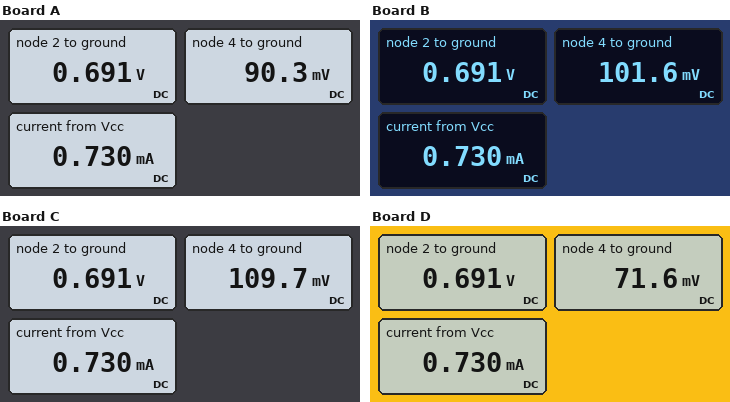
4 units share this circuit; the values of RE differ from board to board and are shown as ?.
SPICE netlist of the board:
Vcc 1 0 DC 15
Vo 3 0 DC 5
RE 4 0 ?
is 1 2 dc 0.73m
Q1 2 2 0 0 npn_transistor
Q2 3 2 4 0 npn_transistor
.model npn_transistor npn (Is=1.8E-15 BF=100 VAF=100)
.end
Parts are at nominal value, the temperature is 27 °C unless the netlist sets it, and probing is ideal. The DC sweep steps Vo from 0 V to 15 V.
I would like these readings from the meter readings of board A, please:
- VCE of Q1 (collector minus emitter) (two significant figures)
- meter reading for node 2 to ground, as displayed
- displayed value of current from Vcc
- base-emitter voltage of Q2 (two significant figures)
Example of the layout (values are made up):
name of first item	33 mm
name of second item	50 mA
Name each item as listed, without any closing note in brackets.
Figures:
VCE of Q1 (collector minus emitter)	690 mV
meter reading for node 2 to ground, as displayed	0.691 V
displayed value of current from Vcc	0.730 mA
base-emitter voltage of Q2	600 mV
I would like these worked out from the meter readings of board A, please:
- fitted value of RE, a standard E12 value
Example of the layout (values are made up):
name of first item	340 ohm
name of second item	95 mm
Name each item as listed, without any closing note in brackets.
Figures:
fitted value of RE, a standard E12 value	3.9 kΩ
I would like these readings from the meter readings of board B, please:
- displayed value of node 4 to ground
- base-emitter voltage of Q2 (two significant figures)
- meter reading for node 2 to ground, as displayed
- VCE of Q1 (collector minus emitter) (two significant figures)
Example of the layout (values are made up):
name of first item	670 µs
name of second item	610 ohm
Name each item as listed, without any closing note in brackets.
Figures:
displayed value of node 4 to ground	101.6 mV
base-emitter voltage of Q2	590 mV
meter reading for node 2 to ground, as displayed	0.691 V
VCE of Q1 (collector minus emitter)	690 mV
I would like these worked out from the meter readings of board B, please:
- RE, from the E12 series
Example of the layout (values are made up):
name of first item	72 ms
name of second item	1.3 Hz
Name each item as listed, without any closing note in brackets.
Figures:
RE, from the E12 series	6.8 kΩ
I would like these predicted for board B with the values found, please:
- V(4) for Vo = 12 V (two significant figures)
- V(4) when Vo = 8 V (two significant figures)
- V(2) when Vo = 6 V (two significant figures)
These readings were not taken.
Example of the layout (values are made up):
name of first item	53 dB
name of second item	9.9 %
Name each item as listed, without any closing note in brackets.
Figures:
V(4) for Vo = 12 V	100 mV
V(4) when Vo = 8 V	100 mV
V(2) when Vo = 6 V	690 mV
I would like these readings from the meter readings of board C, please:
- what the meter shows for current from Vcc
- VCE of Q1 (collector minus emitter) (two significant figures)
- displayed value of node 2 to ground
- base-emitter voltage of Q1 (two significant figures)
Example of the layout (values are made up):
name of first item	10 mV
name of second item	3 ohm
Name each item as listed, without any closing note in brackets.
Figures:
what the meter shows for current from Vcc	0.730 mA
VCE of Q1 (collector minus emitter)	690 mV
displayed value of node 2 to ground	0.691 V
base-emitter voltage of Q1	690 mV
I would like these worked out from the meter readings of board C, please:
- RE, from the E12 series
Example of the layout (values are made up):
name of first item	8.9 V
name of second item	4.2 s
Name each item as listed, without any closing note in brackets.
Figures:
RE, from the E12 series	10 kΩ
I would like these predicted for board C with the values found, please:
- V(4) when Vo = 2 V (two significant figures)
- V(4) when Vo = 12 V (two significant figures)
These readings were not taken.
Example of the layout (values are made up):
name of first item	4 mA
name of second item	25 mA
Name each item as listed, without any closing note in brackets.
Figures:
V(4) when Vo = 2 V	110 mV
V(4) when Vo = 12 V	110 mV
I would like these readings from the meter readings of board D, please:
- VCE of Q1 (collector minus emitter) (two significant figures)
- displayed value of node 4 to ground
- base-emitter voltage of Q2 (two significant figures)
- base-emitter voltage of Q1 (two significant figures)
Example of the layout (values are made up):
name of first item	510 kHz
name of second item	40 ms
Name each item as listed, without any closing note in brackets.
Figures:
VCE of Q1 (collector minus emitter)	690 mV
displayed value of node 4 to ground	71.6 mV
base-emitter voltage of Q2	620 mV
base-emitter voltage of Q1	690 mV
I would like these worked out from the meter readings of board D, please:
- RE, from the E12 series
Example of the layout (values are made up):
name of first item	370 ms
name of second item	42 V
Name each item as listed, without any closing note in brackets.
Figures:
RE, from the E12 series	1.5 kΩ
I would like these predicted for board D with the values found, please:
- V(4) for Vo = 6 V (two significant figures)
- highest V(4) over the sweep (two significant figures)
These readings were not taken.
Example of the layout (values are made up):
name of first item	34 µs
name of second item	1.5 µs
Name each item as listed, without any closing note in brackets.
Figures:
V(4) for Vo = 6 V	72 mV
highest V(4) over the sweep	73 mV
